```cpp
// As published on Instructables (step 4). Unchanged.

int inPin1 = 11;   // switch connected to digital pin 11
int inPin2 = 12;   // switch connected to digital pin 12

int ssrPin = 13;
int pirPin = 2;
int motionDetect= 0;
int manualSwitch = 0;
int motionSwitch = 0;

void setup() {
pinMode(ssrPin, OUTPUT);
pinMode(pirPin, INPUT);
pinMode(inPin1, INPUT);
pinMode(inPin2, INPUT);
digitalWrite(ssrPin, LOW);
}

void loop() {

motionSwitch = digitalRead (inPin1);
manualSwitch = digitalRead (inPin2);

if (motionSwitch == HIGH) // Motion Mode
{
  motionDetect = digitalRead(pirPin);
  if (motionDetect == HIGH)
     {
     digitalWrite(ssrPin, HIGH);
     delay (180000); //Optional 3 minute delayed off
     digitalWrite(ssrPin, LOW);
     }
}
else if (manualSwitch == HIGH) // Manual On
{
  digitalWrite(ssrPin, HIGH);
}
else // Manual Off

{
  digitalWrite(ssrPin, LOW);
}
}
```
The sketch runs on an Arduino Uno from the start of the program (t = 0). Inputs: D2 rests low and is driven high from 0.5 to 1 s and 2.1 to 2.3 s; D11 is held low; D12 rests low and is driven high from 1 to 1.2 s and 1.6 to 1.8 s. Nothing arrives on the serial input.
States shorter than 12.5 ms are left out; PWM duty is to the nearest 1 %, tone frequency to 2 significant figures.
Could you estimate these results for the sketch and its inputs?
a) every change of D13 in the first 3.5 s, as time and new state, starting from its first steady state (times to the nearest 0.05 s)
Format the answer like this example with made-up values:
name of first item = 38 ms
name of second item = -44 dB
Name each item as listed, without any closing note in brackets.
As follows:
every change of D13 in the first 3.5 s, as time and new state, starting from its first steady state = 0 s low; 1 s high; 1.2 s low; 1.6 s high; 1.8 s low
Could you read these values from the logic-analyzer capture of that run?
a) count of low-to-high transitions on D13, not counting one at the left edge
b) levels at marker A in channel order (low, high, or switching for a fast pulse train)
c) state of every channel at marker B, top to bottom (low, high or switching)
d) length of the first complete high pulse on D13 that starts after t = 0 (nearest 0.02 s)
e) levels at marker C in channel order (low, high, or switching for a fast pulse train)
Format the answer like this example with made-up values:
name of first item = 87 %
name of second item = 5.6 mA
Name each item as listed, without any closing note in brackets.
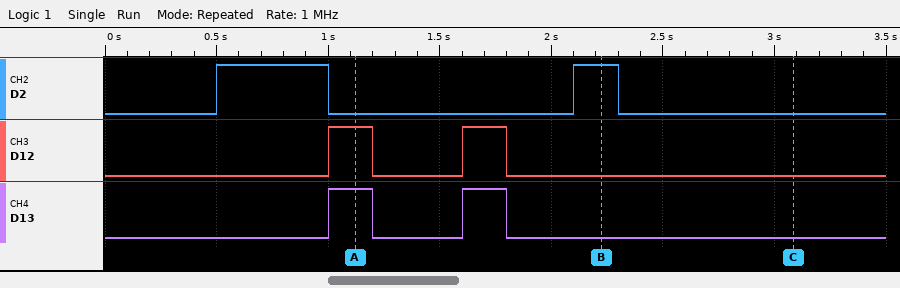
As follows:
count of low-to-high transitions on D13, not counting one at the left edge = 2
levels at marker A in channel order = D2 low, D12 high, D13 high
state of every channel at marker B, top to bottom = D2 high, D12 low, D13 low
length of the first complete high pulse on D13 that starts after t = 0 = 0.20 s
levels at marker C in channel order = D2 low, D12 low, D13 low
